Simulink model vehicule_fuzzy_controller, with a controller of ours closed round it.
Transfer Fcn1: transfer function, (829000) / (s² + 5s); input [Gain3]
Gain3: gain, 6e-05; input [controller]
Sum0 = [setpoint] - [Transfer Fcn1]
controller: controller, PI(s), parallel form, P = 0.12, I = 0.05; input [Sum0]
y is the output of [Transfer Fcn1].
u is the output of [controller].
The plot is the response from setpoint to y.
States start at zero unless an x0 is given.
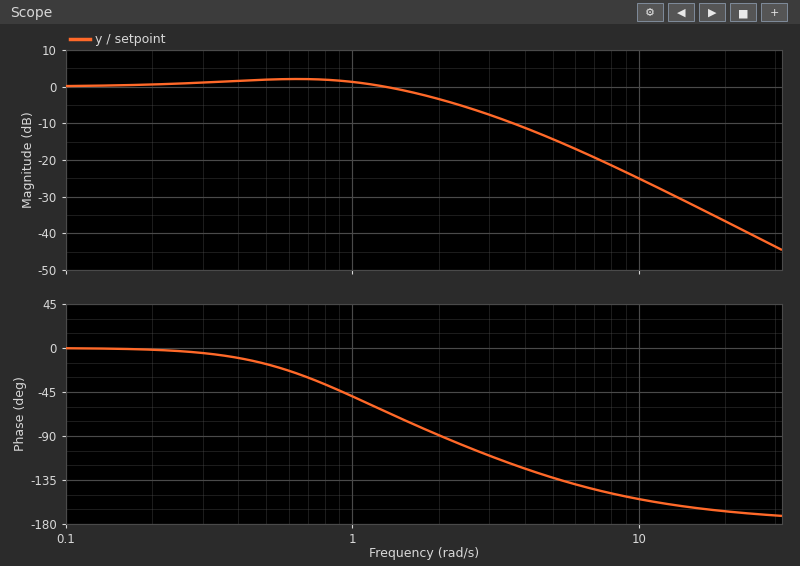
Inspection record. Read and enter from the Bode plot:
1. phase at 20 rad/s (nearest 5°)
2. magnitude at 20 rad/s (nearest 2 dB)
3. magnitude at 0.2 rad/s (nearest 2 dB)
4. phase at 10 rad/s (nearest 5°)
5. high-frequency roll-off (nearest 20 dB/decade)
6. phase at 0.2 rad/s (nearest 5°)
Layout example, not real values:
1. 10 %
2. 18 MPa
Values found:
1. -165°
2. -36 dB
3. 0 dB
4. -155°
5. -40 dB/decade
6. 0°
